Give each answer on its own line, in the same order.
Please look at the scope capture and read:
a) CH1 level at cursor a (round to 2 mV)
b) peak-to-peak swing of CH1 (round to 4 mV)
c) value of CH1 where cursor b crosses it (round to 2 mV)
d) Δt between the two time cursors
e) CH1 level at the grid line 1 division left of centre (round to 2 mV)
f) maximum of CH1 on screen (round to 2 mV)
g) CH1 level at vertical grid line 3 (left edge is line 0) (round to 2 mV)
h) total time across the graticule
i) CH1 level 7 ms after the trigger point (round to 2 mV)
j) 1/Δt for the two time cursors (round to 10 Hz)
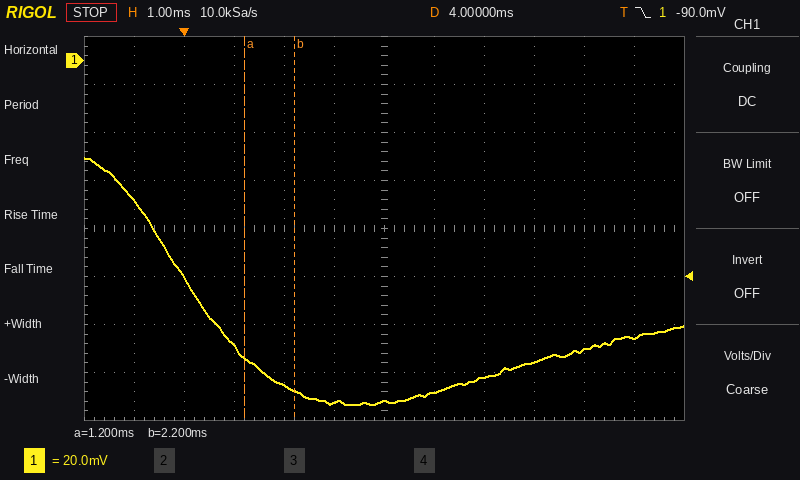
-124 mV
104 mV
-138 mV
1.0 ms
-142 mV
-40 mV
-118 mV
12 ms
-126 mV
1.00 kHz
